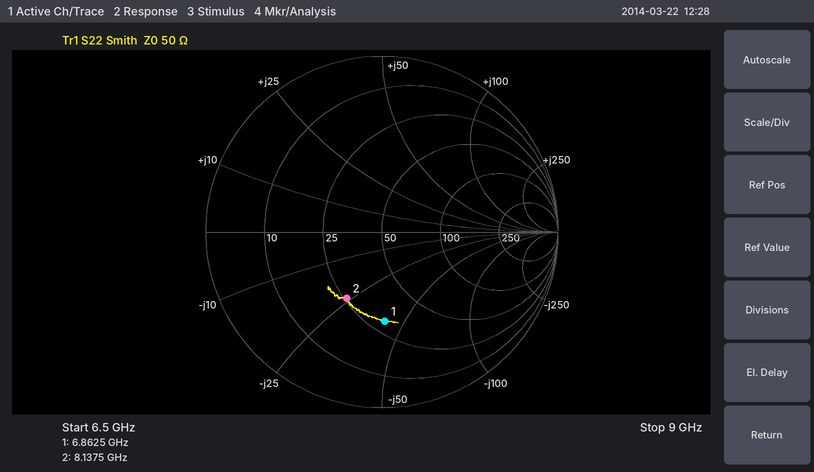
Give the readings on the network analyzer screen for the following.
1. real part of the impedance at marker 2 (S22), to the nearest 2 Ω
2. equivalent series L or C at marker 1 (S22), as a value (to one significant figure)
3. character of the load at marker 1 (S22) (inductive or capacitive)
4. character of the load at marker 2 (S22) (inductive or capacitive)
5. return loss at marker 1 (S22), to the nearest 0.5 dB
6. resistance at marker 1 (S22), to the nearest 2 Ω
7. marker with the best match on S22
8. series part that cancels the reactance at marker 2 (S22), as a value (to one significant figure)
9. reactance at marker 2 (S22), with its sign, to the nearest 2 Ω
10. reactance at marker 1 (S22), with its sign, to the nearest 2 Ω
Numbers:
26 Ω
600 fF
capacitive
capacitive
6.0 dB
30 Ω
marker 2
500 pH
-24 Ω
-42 Ω
